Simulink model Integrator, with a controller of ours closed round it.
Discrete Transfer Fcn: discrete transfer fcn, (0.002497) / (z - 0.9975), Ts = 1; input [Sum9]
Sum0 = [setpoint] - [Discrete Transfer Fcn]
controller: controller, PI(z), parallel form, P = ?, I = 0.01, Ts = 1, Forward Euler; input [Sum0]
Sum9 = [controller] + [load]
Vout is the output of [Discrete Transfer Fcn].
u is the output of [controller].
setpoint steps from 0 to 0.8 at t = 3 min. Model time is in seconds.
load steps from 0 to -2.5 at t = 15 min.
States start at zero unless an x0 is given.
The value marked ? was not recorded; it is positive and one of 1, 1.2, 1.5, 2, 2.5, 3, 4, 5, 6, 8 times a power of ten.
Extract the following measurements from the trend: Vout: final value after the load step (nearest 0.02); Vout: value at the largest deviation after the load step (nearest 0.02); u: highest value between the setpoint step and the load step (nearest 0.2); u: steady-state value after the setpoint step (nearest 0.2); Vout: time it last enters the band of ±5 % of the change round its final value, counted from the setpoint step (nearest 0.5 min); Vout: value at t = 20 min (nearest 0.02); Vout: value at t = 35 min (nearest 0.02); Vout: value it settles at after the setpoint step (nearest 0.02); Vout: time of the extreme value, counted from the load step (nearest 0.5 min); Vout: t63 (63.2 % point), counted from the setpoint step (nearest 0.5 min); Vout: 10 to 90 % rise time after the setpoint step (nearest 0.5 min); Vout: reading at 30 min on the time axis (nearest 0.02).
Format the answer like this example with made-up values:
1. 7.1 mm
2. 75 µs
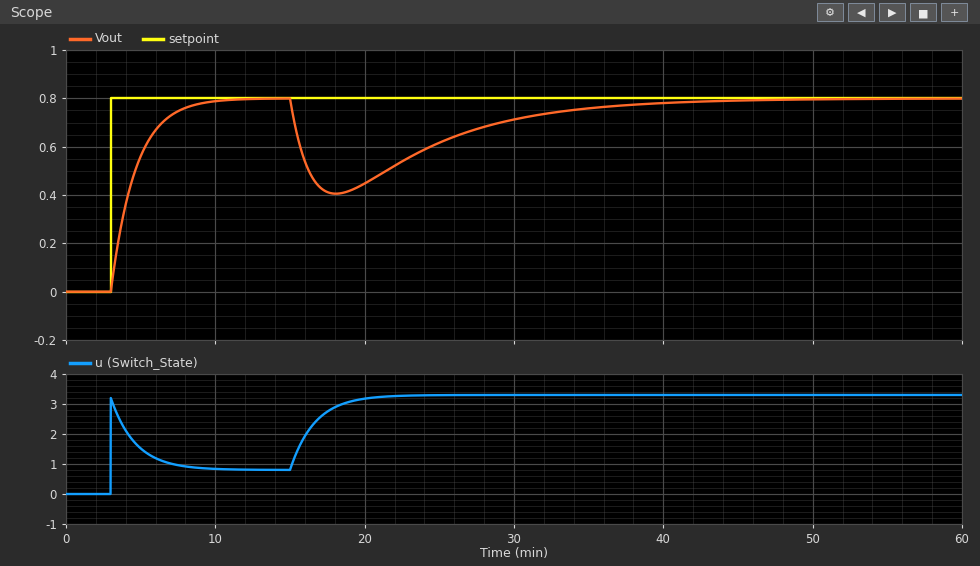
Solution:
1. 0.80
2. 0.40
3. 3.2
4. 0.8
5. 5.0 min
6. 0.44
7. 0.76
8. 0.80
9. 3.0 min
10. 1.5 min
11. 3.5 min
12. 0.72
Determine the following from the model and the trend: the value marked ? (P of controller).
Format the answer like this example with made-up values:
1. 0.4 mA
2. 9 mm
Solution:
1. 4
